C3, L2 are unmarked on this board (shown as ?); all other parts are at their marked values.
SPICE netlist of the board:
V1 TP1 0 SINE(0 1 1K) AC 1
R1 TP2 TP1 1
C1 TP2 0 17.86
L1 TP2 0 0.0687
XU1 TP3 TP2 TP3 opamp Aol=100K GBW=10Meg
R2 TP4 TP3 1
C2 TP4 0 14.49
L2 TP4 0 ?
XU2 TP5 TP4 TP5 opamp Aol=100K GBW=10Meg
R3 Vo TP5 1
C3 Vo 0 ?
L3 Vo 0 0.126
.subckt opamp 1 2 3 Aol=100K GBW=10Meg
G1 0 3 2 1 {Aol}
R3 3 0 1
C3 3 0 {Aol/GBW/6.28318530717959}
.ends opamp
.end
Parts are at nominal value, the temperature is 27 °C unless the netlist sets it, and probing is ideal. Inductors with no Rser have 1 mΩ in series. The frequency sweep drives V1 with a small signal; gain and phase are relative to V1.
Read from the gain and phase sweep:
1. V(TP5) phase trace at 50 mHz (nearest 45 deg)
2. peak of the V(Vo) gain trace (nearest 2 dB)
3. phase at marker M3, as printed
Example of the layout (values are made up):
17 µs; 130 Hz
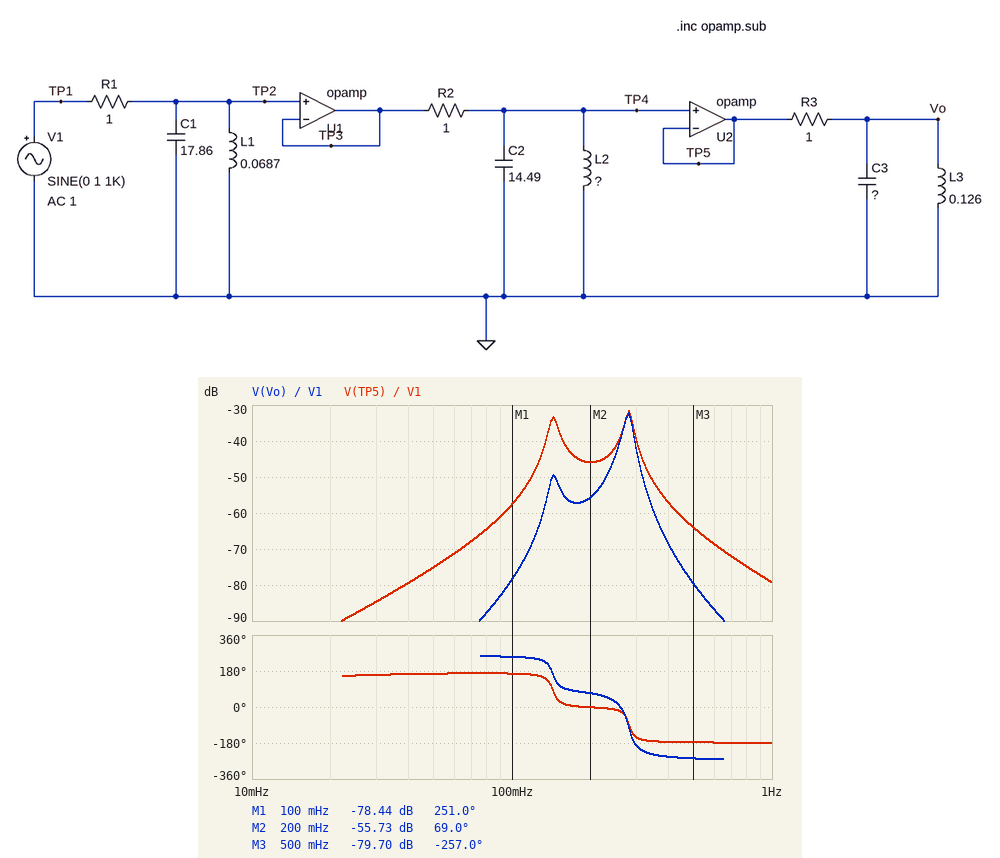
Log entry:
180 deg; -32 dB; -257.0 deg
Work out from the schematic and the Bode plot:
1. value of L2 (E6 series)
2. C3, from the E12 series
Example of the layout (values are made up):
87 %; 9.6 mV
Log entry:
22 mH; 2.7 F
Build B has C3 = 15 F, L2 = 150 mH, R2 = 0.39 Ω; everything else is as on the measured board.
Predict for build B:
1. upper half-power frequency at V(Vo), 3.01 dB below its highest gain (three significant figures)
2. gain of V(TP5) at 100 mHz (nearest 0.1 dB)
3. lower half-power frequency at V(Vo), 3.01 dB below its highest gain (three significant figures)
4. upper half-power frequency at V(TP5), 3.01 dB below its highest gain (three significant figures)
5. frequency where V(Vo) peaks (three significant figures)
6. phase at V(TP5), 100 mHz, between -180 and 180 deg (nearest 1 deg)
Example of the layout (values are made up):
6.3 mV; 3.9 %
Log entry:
123 mHz; -23.2 dB; 111 mHz; 148 mHz; 116 mHz; 112 deg
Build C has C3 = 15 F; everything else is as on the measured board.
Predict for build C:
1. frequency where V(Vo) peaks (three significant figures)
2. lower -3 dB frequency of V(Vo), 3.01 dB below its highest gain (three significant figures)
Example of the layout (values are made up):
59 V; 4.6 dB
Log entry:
143 mHz; 136 mHz
